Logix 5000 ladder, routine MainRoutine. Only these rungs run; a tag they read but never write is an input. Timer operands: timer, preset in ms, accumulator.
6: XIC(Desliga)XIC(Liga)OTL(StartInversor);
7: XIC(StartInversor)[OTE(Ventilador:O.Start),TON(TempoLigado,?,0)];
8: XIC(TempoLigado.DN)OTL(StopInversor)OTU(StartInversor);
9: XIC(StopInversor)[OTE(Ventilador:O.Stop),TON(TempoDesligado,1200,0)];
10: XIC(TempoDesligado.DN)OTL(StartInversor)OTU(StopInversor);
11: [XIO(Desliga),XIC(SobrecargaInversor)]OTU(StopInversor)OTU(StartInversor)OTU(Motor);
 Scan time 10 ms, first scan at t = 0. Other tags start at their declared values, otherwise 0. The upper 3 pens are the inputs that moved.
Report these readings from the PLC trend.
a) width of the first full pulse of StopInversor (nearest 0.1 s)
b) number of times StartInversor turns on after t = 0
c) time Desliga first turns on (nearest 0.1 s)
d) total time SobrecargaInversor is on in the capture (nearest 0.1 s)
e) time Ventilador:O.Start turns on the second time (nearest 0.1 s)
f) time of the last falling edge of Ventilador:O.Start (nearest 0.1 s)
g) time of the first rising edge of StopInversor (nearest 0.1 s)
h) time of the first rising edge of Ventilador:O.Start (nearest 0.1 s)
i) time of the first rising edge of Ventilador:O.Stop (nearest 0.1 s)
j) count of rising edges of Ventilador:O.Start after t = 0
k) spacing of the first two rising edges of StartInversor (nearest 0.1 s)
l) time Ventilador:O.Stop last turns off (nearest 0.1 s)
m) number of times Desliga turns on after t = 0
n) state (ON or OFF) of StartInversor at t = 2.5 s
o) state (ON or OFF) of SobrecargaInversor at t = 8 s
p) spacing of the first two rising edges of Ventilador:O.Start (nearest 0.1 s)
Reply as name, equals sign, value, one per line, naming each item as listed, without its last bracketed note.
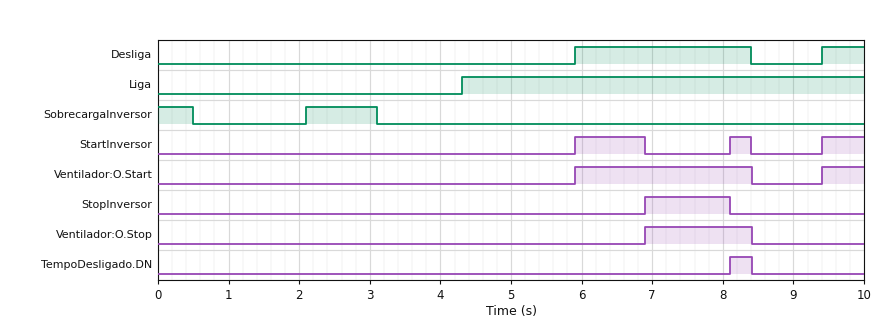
width of the first full pulse of StopInversor = 1.2 s
number of times StartInversor turns on after t = 0 = 3
time Desliga first turns on = 5.9 s
total time SobrecargaInversor is on in the capture = 1.5 s
time Ventilador:O.Start turns on the second time = 9.4 s
time of the last falling edge of Ventilador:O.Start = 8.4 s
time of the first rising edge of StopInversor = 6.9 s
time of the first rising edge of Ventilador:O.Start = 5.9 s
time of the first rising edge of Ventilador:O.Stop = 6.9 s
count of rising edges of Ventilador:O.Start after t = 0 = 2
spacing of the first two rising edges of StartInversor = 2.2 s
time Ventilador:O.Stop last turns off = 8.4 s
number of times Desliga turns on after t = 0 = 2
state (ON or OFF) of StartInversor at t = 2.5 s = OFF
state (ON or OFF) of SobrecargaInversor at t = 8 s = OFF
spacing of the first two rising edges of Ventilador:O.Start = 3.5 s
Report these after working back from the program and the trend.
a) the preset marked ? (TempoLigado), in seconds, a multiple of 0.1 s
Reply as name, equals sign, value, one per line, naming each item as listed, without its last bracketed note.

the preset marked ? (TempoLigado), in seconds, a multiple of 0.1 s = 1.0 s
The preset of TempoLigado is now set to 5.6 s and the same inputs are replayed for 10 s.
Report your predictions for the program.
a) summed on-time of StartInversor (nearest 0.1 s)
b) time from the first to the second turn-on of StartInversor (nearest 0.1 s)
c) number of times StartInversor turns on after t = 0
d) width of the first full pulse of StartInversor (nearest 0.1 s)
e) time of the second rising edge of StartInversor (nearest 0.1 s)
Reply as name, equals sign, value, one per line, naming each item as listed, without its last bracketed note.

summed on-time of StartInversor = 3.1 s
time from the first to the second turn-on of StartInversor = 3.5 s
number of times StartInversor turns on after t = 0 = 2
width of the first full pulse of StartInversor = 2.5 s
time of the second rising edge of StartInversor = 9.4 s
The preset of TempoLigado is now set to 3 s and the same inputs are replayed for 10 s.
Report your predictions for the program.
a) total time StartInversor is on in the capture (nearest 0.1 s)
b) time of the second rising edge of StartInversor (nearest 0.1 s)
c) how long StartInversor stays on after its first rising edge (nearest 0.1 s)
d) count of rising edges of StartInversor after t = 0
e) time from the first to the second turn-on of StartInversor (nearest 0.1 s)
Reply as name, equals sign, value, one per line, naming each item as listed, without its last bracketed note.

total time StartInversor is on in the capture = 3.1 s
time of the second rising edge of StartInversor = 9.4 s
how long StartInversor stays on after its first rising edge = 2.5 s
count of rising edges of StartInversor after t = 0 = 2
time from the first to the second turn-on of StartInversor = 3.5 s
